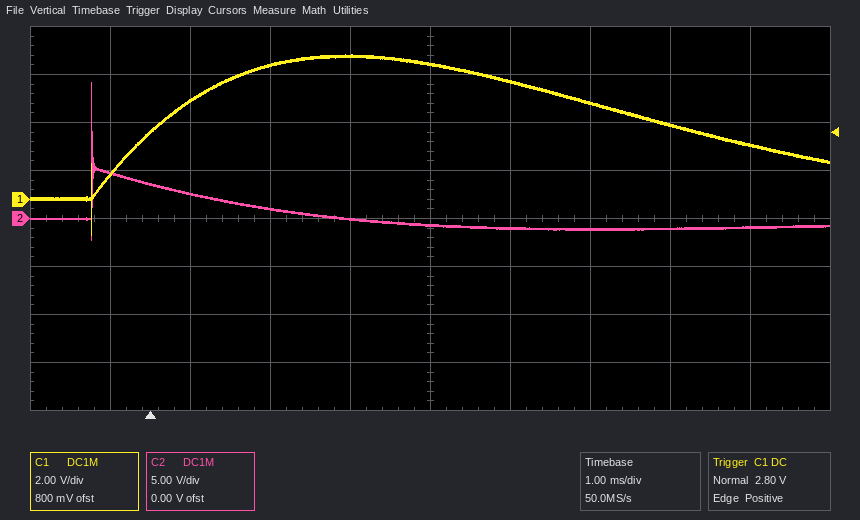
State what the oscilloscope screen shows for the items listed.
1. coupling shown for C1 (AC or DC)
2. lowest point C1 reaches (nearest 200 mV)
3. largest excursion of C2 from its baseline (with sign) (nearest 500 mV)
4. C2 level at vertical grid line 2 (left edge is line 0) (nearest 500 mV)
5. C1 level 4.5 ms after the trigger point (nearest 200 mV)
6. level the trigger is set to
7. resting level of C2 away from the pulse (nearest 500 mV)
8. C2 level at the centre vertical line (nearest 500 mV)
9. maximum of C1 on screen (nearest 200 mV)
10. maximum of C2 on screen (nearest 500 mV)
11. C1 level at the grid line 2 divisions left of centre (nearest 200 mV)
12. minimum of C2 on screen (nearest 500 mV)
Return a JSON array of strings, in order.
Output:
["DC", "-1.4 V", "+15.0 V", "2.5 V", "5.0 V", "2.80 V", "-1.0 V", "-500 mV", "6.0 V", "14.0 V", "5.6 V", "-2.0 V"]
